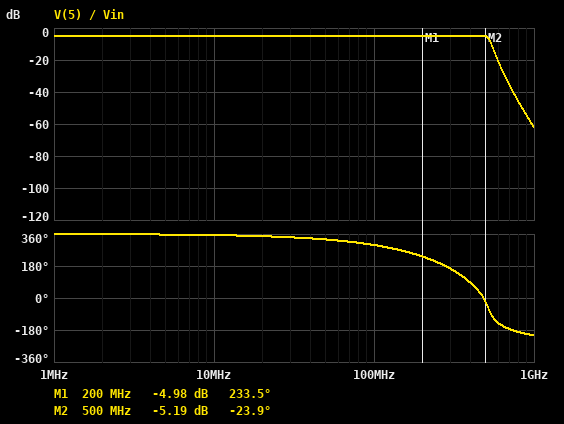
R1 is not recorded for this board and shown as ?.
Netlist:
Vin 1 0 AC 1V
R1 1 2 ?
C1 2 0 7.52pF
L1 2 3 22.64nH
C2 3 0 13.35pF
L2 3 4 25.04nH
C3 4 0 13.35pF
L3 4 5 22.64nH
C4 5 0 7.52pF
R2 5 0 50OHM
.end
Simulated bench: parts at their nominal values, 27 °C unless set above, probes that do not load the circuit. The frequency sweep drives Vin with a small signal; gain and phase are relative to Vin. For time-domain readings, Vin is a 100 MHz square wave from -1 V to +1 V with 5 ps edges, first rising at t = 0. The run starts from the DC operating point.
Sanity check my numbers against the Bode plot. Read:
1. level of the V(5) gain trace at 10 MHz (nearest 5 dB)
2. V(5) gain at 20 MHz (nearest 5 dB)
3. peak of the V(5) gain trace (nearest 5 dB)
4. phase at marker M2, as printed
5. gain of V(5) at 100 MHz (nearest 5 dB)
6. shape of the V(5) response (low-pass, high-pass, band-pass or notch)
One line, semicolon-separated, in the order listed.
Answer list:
-5 dB; -5 dB; -5 dB; -23.9 deg; -5 dB; low-pass
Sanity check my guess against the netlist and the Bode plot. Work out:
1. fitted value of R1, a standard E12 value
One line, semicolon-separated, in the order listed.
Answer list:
39 Ω
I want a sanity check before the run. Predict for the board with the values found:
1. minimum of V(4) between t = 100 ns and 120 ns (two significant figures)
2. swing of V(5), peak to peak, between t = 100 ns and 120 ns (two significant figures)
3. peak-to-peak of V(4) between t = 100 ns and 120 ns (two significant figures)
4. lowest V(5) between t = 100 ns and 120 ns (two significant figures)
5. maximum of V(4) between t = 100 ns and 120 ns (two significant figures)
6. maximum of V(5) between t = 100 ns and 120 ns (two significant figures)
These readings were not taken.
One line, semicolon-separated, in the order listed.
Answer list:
-790 mV; 1.6 V; 1.6 V; -800 mV; 790 mV; 800 mV
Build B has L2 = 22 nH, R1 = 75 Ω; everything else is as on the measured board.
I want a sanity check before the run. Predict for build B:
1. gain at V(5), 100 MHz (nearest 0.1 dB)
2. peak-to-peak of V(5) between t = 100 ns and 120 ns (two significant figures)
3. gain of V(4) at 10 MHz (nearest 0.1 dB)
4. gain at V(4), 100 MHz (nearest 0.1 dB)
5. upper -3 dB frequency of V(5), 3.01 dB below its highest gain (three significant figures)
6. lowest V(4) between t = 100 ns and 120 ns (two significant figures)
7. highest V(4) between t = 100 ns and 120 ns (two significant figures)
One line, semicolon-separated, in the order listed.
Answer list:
-8.3 dB; 1.1 V; -8.0 dB; -8.6 dB; 560 MHz; -530 mV; 530 mV
